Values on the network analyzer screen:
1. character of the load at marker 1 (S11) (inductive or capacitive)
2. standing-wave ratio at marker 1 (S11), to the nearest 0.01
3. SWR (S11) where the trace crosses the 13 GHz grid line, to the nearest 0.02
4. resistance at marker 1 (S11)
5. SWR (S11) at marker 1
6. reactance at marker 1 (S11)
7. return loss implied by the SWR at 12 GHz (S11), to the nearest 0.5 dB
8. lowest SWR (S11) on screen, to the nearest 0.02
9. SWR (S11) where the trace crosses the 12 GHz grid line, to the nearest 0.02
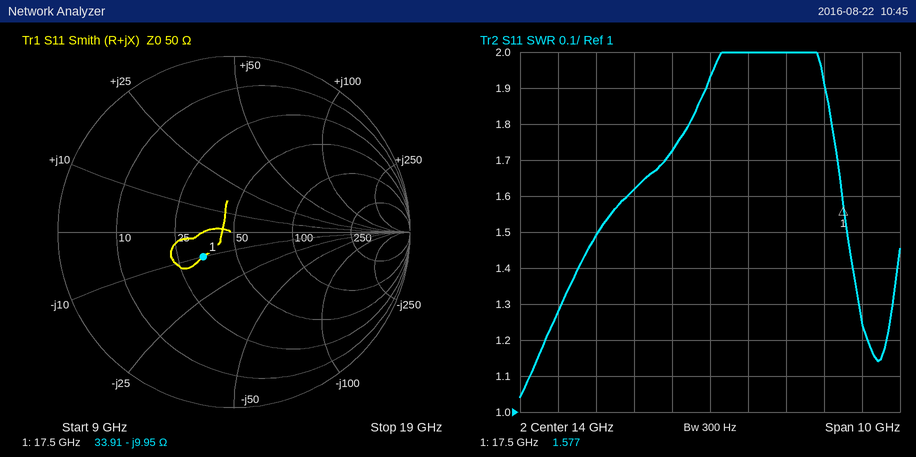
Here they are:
capacitive
1.58
1.72
33.91 Ω
1.577
-9.95 Ω
12.5 dB
1.04
1.62
